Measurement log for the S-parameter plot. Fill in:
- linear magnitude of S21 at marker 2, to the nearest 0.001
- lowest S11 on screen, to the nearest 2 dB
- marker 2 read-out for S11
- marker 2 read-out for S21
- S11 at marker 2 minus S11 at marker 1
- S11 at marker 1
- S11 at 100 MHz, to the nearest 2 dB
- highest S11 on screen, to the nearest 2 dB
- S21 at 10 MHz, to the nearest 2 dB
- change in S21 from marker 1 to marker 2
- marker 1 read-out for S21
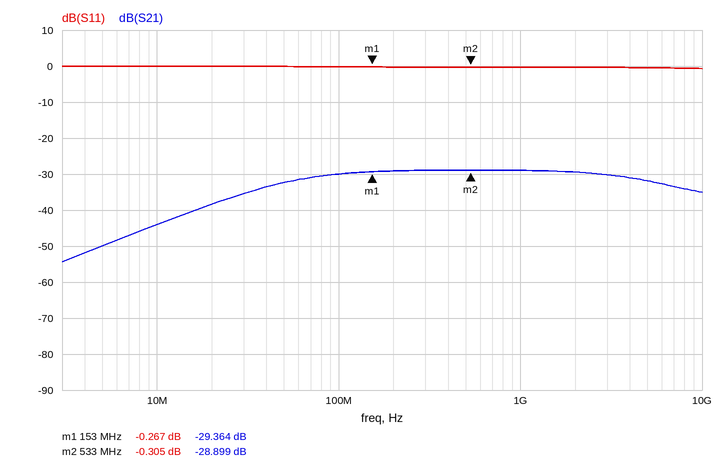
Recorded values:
0.036
0 dB
-0.305 dB
-28.899 dB
-0.038 dB
-0.267 dB
0 dB
0 dB
-44 dB
0.465 dB
-29.364 dB
